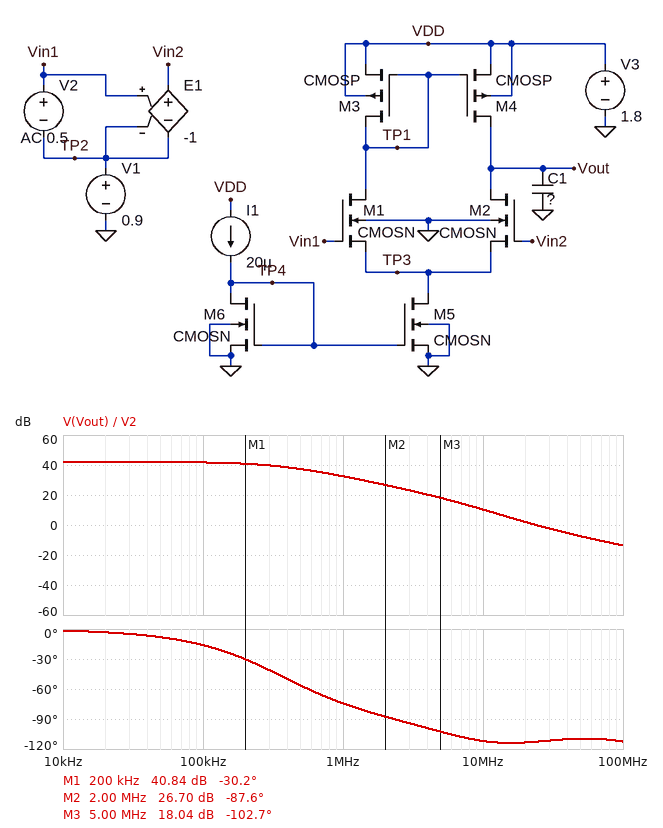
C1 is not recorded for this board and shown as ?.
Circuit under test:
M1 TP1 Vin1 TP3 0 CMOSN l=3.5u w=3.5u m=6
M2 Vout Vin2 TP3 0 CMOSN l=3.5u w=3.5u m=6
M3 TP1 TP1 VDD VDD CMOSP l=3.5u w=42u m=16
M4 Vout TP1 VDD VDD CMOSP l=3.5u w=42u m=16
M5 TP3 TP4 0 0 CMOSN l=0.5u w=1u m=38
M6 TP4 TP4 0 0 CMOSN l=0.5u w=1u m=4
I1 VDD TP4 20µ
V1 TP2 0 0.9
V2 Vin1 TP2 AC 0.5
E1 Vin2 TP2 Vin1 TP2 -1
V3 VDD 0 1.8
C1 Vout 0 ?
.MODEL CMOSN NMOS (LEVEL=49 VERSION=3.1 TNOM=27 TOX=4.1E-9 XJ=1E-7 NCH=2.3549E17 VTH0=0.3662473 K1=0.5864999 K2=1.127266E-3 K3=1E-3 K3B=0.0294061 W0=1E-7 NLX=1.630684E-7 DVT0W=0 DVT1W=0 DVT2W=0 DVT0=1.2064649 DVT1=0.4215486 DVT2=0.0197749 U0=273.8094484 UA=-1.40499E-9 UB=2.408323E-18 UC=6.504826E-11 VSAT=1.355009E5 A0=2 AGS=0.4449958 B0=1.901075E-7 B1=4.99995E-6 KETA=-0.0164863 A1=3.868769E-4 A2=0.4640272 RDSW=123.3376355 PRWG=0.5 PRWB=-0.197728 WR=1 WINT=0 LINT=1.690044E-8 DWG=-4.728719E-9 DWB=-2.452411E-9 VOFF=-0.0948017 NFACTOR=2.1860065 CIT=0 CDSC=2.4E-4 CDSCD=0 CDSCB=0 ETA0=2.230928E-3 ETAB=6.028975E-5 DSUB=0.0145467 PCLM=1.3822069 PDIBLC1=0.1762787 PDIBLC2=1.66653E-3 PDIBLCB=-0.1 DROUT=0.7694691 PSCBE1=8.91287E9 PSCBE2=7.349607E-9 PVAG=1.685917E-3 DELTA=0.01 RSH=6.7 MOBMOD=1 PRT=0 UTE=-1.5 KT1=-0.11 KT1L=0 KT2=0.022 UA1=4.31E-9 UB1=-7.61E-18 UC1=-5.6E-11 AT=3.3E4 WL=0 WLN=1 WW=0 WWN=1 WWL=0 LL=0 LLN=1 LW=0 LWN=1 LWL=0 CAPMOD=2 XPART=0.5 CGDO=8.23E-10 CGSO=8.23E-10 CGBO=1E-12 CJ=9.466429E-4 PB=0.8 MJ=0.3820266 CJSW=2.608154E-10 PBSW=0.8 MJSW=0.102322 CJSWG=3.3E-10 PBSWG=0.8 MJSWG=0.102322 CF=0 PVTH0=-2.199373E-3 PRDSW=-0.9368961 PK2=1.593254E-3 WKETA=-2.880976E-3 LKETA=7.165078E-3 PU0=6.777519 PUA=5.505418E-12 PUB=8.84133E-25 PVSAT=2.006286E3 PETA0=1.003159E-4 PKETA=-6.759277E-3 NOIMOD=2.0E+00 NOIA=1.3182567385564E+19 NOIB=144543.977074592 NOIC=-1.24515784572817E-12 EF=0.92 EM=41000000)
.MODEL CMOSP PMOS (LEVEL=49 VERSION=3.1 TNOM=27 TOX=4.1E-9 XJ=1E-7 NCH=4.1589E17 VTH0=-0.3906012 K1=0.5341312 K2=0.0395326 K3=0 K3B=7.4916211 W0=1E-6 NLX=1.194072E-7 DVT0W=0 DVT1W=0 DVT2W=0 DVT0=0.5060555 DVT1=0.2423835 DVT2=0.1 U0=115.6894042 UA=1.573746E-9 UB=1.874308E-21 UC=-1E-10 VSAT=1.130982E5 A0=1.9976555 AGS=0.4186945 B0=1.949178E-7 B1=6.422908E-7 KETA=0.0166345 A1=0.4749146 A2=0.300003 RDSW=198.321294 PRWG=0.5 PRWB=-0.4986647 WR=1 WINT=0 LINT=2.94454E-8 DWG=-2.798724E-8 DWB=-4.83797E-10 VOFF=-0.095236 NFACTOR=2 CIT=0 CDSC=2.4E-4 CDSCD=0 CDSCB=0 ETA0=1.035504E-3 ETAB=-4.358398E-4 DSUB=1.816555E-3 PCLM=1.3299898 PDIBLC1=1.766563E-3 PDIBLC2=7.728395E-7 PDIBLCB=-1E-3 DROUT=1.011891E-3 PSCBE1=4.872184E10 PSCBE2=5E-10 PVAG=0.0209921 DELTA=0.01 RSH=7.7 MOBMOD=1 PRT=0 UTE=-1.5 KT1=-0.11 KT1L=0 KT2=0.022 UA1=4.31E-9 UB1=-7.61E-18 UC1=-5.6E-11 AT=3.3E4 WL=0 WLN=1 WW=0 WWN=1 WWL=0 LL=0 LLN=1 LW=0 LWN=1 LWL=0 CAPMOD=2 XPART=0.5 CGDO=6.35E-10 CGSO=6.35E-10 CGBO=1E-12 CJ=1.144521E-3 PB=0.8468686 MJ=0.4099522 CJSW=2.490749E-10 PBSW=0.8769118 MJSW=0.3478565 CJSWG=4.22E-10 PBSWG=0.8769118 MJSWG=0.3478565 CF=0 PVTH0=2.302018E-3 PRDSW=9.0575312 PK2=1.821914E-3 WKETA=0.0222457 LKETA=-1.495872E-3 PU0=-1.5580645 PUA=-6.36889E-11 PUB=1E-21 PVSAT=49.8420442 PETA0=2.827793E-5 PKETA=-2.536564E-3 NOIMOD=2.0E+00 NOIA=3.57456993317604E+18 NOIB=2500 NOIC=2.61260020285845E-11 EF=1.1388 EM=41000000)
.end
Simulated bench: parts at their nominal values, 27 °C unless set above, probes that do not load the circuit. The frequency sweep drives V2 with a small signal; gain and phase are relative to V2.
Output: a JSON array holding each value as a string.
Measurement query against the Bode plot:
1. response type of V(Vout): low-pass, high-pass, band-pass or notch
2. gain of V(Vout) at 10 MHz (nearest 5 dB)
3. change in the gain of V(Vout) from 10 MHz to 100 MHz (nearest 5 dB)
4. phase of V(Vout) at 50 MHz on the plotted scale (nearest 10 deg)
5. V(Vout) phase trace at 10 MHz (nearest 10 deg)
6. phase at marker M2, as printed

["low-pass", "10 dB", "-25 dB", "-110 deg", "-110 deg", "-87.6 deg"]
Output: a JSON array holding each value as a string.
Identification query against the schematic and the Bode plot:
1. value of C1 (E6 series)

["2.2 pF"]
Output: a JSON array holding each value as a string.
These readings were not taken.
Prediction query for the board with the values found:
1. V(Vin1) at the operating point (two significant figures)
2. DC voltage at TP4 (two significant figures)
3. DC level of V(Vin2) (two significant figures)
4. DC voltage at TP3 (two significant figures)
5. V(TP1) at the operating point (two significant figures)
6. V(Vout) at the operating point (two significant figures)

["900 mV", "570 mV", "900 mV", "130 mV", "1.3 V", "1.3 V"]
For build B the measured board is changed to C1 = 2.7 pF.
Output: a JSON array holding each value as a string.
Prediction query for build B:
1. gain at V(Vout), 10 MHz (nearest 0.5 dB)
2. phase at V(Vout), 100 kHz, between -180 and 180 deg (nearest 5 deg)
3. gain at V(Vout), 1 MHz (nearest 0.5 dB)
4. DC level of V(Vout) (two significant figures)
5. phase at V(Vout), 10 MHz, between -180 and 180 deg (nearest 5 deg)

["9.0 dB", "-20 deg", "31.5 dB", "1.3 V", "-115 deg"]
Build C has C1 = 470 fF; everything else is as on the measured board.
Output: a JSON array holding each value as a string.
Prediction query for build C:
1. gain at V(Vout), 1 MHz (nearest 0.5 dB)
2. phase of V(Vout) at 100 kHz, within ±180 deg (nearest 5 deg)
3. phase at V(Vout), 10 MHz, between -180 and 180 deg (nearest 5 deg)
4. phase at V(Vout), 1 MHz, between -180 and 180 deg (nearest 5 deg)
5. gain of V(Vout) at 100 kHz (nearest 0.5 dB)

["37.5 dB", "-10 deg", "-105 deg", "-55 deg", "42.0 dB"]
